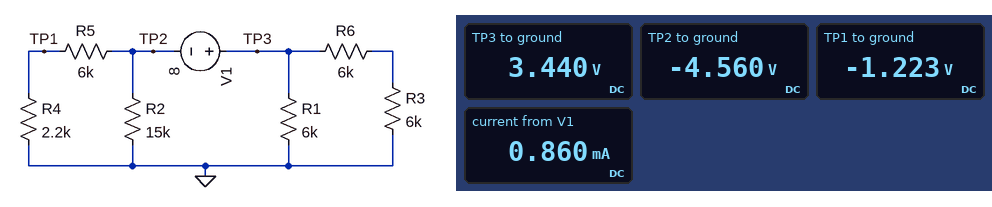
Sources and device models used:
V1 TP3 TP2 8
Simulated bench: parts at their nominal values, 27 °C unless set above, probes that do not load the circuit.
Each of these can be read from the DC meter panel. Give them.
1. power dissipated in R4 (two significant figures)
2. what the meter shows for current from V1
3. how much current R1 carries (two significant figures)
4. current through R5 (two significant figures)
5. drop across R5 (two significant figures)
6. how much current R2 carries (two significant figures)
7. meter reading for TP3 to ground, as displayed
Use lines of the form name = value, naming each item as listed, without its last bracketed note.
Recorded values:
power dissipated in R4 = 680 µW
what the meter shows for current from V1 = 0.860 mA
how much current R1 carries = 570 µA
current through R5 = 560 µA
drop across R5 = 3.3 V
how much current R2 carries = 300 µA
meter reading for TP3 to ground, as displayed = 3.440 V
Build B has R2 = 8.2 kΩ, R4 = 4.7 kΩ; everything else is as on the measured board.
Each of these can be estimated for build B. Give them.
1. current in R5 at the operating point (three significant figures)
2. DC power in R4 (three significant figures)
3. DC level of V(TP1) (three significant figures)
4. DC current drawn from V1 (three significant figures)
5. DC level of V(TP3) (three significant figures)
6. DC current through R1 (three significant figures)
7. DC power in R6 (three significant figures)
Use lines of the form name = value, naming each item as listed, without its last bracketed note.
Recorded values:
current in R5 at the operating point = 402 µA
DC power in R4 = 758 µW
DC level of V(TP1) = -1.89 V
DC current drawn from V1 = 926 µA
DC level of V(TP3) = 3.70 V
DC current through R1 = 617 µA
DC power in R6 = 571 µW
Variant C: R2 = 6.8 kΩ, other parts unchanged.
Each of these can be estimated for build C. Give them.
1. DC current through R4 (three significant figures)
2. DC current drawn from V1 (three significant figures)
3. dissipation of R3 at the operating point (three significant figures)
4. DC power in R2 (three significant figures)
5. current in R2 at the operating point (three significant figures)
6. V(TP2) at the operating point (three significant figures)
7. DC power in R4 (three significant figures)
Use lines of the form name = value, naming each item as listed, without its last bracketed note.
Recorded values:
DC current through R4 = 470 µA
DC current drawn from V1 = 1.04 mA
dissipation of R3 at the operating point = 716 µW
DC power in R2 = 2.18 mW
current in R2 at the operating point = 567 µA
V(TP2) at the operating point = -3.85 V
DC power in R4 = 486 µW
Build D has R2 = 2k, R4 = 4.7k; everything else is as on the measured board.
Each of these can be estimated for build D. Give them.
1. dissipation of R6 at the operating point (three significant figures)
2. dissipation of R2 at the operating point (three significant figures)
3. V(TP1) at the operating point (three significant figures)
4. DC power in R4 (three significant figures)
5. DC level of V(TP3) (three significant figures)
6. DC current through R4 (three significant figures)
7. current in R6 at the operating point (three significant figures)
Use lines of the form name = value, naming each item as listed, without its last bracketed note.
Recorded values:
dissipation of R6 at the operating point = 1.32 mW
dissipation of R2 at the operating point = 2.81 mW
V(TP1) at the operating point = -1.04 V
DC power in R4 = 231 µW
DC level of V(TP3) = 5.63 V
DC current through R4 = 222 µA
current in R6 at the operating point = 469 µA
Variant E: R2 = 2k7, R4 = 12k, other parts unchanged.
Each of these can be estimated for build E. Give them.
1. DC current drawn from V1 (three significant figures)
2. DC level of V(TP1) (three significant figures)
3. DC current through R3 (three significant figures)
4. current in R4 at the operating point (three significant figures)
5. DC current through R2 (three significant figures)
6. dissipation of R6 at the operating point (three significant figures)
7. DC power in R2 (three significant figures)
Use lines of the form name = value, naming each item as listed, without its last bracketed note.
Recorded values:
DC current drawn from V1 = 1.26 mA
DC level of V(TP1) = -1.97 V
DC current through R3 = 420 µA
current in R4 at the operating point = 164 µA
DC current through R2 = 1.10 mA
dissipation of R6 at the operating point = 1.06 mW
DC power in R2 = 3.24 mW
